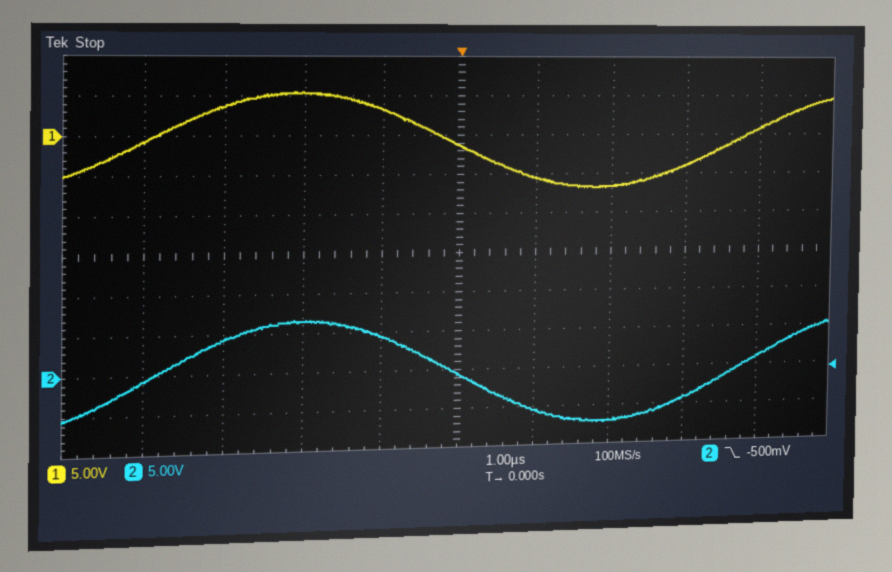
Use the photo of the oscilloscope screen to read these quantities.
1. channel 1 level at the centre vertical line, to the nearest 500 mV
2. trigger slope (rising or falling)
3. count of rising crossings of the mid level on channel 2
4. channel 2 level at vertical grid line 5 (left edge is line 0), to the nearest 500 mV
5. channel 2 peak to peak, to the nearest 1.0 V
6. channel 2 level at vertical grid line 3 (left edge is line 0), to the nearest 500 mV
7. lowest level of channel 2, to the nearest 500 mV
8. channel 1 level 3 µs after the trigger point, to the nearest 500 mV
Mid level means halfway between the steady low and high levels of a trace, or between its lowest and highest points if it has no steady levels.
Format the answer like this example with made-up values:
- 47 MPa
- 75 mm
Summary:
- -1.5 V
- falling
- 2
- -500 mV
- 14.0 V
- 6.5 V
- -7.0 V
- -4.0 V
